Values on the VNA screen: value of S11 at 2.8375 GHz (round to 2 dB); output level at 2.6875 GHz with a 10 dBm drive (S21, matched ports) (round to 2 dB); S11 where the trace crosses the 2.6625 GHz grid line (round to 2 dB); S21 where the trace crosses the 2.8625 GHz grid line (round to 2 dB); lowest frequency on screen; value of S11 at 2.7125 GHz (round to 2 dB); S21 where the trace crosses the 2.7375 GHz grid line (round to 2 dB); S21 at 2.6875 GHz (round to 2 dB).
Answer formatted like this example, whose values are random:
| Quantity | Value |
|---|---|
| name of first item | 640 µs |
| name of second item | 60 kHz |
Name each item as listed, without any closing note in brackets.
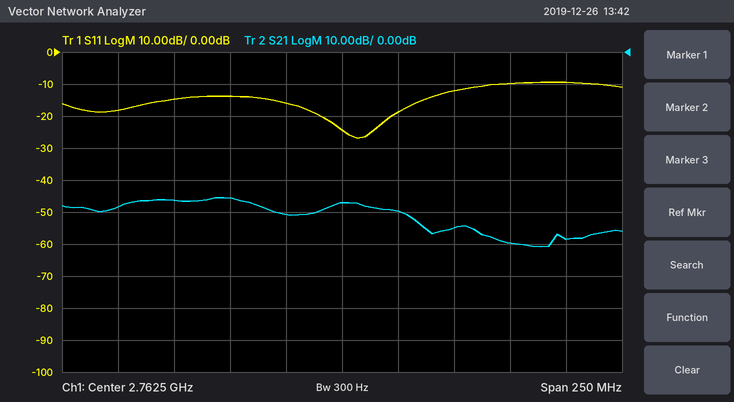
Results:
| Quantity | Value |
|---|---|
| value of S11 at 2.8375 GHz | -10 dB |
| output level at 2.6875 GHz with a 10 dBm drive (S21, matched ports) | -36 dBm |
| S11 where the trace crosses the 2.6625 GHz grid line | -18 dB |
| S21 where the trace crosses the 2.8625 GHz grid line | -58 dB |
| lowest frequency on screen | 2.6375 GHz |
| value of S11 at 2.7125 GHz | -14 dB |
| S21 where the trace crosses the 2.7375 GHz grid line | -50 dB |
| S21 at 2.6875 GHz | -46 dB |
